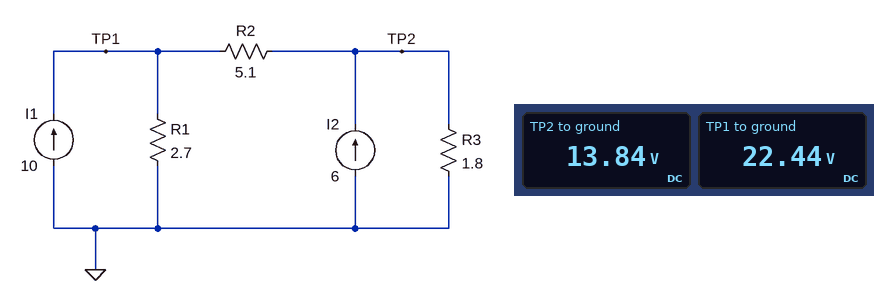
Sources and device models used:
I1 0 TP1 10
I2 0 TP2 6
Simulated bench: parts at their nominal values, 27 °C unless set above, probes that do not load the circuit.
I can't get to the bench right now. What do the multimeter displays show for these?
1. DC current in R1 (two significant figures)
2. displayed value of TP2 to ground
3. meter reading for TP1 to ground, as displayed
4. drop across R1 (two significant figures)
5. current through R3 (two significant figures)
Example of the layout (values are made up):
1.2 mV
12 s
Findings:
8.3 A
13.84 V
22.44 V
22 V
7.7 A
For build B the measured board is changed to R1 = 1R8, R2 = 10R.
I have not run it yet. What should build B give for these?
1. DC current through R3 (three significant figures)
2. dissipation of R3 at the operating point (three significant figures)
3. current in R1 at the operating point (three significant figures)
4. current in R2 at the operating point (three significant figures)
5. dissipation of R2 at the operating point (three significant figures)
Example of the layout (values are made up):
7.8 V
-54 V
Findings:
6.53 A
76.7 W
9.47 A
529 mA
2.80 W
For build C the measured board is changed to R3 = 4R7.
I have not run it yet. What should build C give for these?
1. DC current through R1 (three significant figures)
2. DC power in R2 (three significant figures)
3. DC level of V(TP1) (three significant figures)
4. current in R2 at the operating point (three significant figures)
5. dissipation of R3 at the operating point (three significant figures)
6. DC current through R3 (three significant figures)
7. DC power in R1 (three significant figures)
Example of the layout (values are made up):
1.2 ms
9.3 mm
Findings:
10.1 A
47.0 mW
27.3 V
96.0 mA
164 W
5.90 A
275 W
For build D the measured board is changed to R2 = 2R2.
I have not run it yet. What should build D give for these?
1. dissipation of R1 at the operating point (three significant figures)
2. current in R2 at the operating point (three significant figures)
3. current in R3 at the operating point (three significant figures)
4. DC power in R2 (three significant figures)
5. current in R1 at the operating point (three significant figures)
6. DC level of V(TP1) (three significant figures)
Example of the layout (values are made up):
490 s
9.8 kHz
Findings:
155 W
2.42 A
8.42 A
12.9 W
7.58 A
20.5 V
